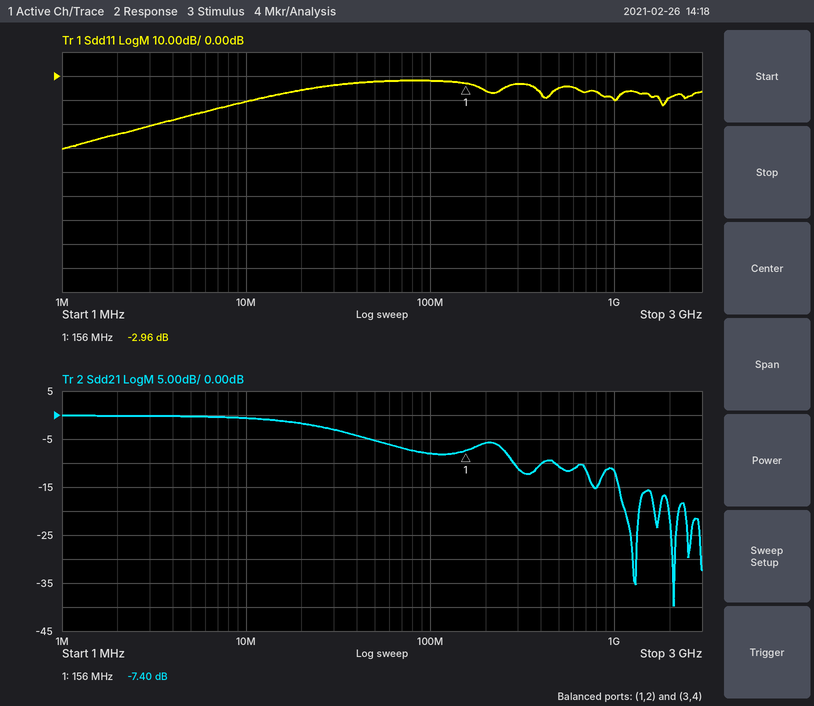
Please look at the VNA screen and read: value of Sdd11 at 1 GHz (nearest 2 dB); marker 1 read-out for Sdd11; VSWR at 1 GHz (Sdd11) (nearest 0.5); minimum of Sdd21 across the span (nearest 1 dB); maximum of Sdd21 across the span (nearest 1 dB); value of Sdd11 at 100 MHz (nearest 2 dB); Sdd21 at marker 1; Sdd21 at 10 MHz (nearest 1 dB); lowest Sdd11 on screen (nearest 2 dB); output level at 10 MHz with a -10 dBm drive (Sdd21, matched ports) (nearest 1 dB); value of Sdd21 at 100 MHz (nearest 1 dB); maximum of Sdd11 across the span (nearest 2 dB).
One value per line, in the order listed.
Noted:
-10 dB
-2.96 dB
2.0
-40 dB
0 dB
-2 dB
-7.40 dB
-1 dB
-30 dB
-11 dBm
-8 dB
-2 dB
